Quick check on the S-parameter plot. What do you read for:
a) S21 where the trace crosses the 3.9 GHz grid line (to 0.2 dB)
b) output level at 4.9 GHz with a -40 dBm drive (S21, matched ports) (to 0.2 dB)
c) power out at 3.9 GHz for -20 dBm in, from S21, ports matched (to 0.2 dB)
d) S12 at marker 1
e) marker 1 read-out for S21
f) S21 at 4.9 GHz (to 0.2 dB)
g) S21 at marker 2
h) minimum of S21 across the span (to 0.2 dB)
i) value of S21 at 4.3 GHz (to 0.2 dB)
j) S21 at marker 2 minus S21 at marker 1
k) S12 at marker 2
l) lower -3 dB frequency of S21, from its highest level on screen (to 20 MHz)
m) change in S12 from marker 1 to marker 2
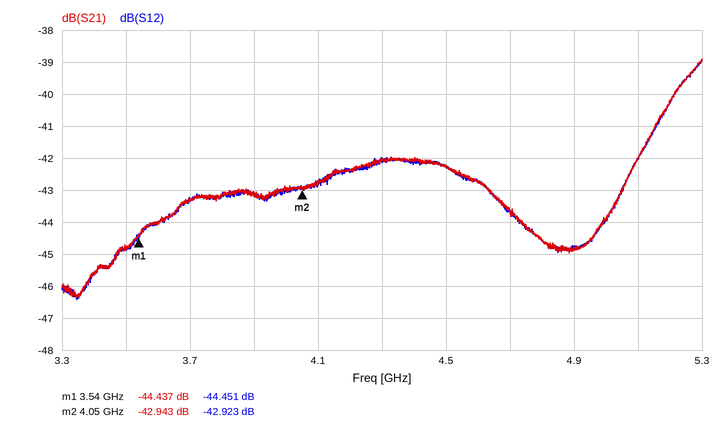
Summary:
-43.2 dB
-84.8 dBm
-63.2 dBm
-44.451 dB
-44.437 dB
-44.8 dB
-42.943 dB
-46.4 dB
-42.0 dB
1.494 dB
-42.923 dB
5.10 GHz
1.528 dB
